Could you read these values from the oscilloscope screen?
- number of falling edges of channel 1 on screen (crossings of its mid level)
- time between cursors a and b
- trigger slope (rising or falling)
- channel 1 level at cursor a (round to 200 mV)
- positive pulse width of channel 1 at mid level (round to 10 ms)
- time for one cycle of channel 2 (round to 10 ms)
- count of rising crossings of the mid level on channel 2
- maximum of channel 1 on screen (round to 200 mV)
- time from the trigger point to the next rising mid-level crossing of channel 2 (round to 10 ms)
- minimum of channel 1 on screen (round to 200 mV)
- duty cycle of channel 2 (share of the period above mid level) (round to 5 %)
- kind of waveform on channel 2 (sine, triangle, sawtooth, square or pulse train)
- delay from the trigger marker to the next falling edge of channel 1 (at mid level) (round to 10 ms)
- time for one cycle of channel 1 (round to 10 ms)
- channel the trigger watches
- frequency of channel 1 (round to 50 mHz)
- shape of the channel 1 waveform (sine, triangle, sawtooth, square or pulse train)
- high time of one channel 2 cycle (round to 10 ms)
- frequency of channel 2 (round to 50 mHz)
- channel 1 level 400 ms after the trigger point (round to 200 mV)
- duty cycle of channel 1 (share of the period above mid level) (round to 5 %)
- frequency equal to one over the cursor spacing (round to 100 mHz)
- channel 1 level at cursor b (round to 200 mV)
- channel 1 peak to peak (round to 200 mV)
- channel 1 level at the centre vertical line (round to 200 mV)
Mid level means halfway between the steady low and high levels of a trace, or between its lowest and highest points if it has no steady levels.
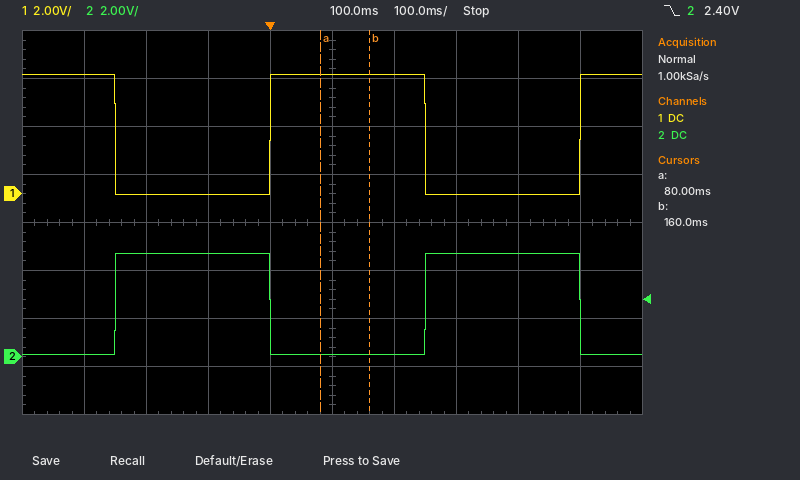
2
80 ms
falling
5.0 V
250 ms
500 ms
2
5.0 V
250 ms
0.0 V
50 %
square
250 ms
500 ms
channel 2
2.00 Hz
square
250 ms
2.00 Hz
0.0 V
50 %
12.5 Hz
5.0 V
5.0 V
5.0 V
